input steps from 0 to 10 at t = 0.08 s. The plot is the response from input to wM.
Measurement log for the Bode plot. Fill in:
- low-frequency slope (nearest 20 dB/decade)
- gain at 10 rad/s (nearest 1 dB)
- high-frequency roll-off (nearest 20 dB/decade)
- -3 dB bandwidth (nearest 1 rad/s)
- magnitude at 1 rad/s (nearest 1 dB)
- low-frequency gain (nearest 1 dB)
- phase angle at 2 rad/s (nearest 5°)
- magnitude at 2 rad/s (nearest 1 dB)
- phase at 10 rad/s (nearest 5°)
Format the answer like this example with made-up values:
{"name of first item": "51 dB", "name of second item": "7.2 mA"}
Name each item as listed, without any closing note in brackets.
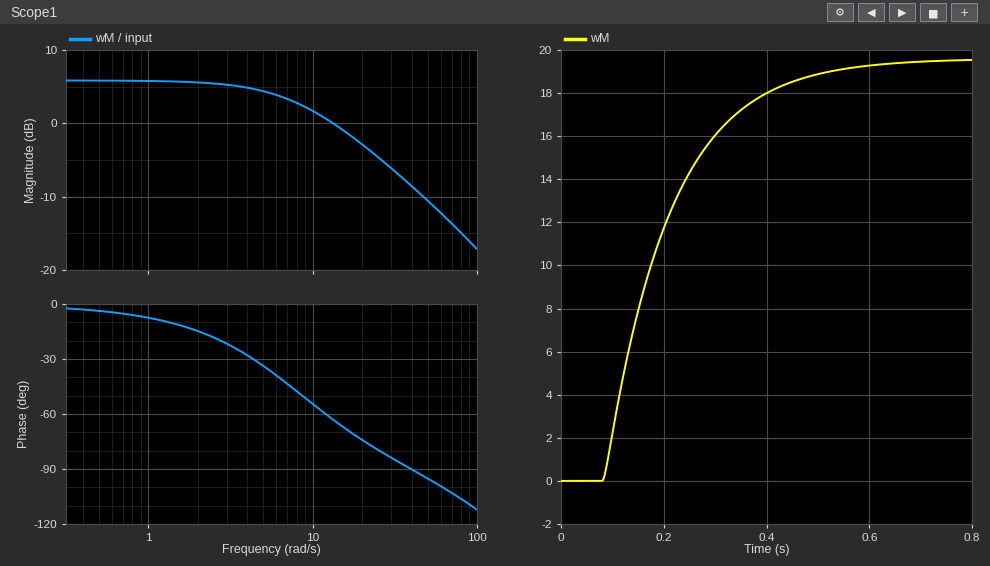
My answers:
{"low-frequency slope": "0 dB/decade", "gain at 10 rad/s": "2 dB", "high-frequency roll-off": "-20 dB/decade", "-3 dB bandwidth": "8 rad/s", "magnitude at 1 rad/s": "6 dB", "low-frequency gain": "6 dB", "phase angle at 2 rad/s": "-15°", "magnitude at 2 rad/s": "6 dB", "phase at 10 rad/s": "-55°"}
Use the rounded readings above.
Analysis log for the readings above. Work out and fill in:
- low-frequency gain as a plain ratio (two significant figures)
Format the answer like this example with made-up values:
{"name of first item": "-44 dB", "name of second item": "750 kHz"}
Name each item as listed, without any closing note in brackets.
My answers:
{"low-frequency gain as a plain ratio": "2.0"}
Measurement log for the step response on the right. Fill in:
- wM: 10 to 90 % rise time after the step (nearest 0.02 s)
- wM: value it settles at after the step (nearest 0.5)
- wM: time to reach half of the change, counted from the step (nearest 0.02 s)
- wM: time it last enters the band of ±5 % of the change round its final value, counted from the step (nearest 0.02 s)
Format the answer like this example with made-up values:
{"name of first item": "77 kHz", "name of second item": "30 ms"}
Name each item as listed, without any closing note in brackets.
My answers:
{"wM: 10 to 90 % rise time after the step": "0.28 s", "wM: value it settles at after the step": "19.5", "wM: time to reach half of the change, counted from the step": "0.10 s", "wM: time it last enters the band of ±5 % of the change round its final value, counted from the step": "0.38 s"}
